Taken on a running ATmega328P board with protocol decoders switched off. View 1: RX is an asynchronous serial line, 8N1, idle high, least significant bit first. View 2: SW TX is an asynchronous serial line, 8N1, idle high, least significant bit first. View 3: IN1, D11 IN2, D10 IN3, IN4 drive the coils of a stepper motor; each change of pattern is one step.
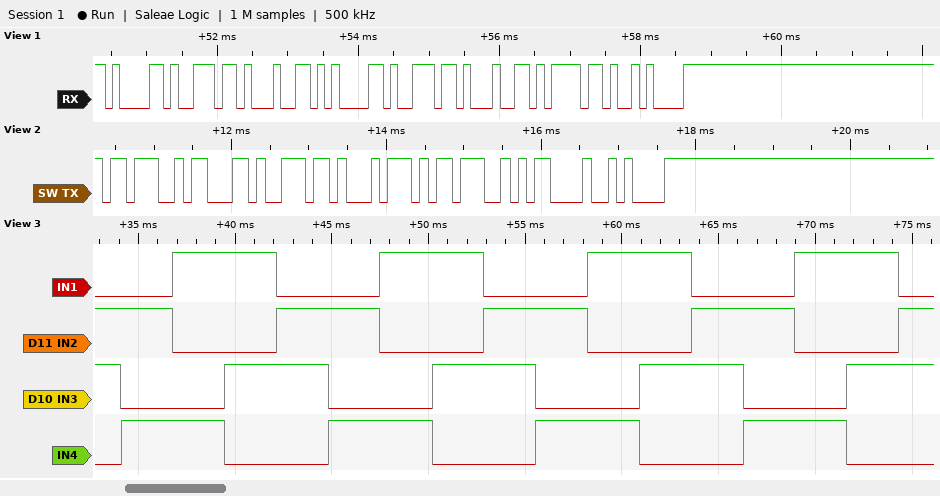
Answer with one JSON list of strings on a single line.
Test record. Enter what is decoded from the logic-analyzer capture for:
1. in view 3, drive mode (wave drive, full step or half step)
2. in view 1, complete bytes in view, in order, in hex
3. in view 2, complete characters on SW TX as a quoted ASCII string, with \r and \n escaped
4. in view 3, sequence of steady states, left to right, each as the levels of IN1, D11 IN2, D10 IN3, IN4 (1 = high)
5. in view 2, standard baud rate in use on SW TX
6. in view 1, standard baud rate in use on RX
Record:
["full step", "61 6E 64 61 6E 64 6F 0A", "\";cnt;\\r\\n\"", "0110 0101 1001 1010 0110 0101 1001 1010 0110 0101 1001 1010 0110 0101 1001 1010 0110", "9600 baud", "9600 baud"]
